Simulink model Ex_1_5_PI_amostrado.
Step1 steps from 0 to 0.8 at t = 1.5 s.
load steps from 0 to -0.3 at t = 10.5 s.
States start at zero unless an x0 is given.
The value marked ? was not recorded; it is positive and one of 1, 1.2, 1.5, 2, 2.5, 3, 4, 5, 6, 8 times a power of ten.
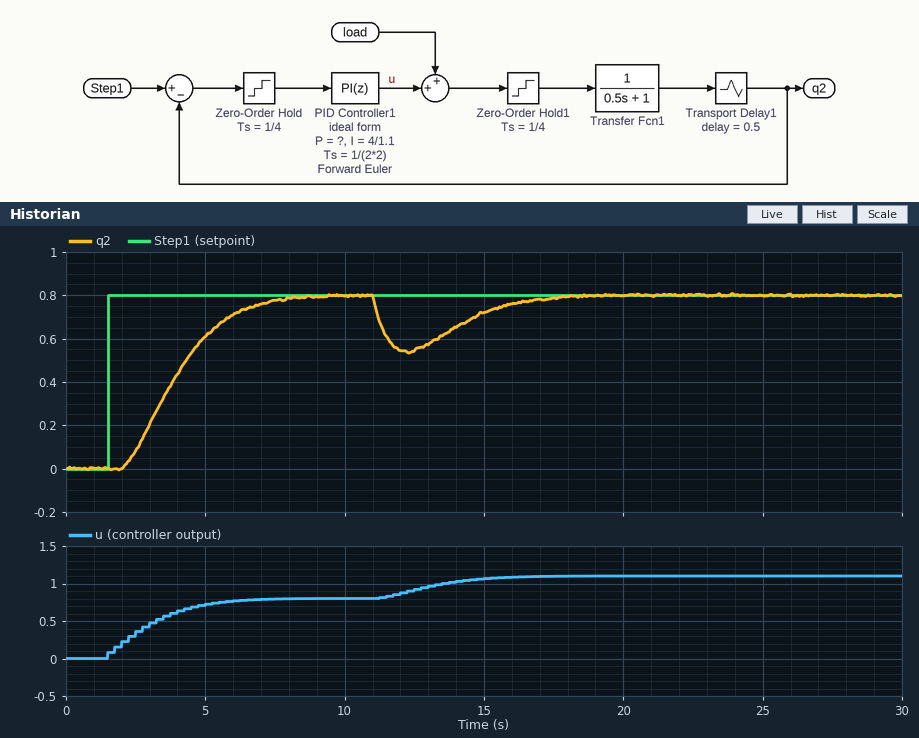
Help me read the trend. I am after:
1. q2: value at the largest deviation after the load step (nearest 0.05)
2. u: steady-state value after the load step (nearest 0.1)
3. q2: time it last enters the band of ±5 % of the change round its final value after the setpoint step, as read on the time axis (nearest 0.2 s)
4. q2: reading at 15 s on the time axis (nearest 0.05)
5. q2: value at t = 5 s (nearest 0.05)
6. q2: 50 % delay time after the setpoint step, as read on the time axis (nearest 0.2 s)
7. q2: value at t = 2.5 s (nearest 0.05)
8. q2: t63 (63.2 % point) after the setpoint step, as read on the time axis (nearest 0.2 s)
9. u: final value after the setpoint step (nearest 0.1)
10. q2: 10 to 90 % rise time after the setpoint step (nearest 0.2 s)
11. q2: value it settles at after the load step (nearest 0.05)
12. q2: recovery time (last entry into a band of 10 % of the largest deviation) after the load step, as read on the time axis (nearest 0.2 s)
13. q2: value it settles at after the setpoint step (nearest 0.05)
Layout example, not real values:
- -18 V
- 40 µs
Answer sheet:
- 0.55
- 1.1
- 7.0 s
- 0.70
- 0.60
- 3.8 s
- 0.10
- 4.4 s
- 0.8
- 3.6 s
- 0.80
- 16.6 s
- 0.80
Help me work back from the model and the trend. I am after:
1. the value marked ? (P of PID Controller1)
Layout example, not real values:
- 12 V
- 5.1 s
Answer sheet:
- 0.1
